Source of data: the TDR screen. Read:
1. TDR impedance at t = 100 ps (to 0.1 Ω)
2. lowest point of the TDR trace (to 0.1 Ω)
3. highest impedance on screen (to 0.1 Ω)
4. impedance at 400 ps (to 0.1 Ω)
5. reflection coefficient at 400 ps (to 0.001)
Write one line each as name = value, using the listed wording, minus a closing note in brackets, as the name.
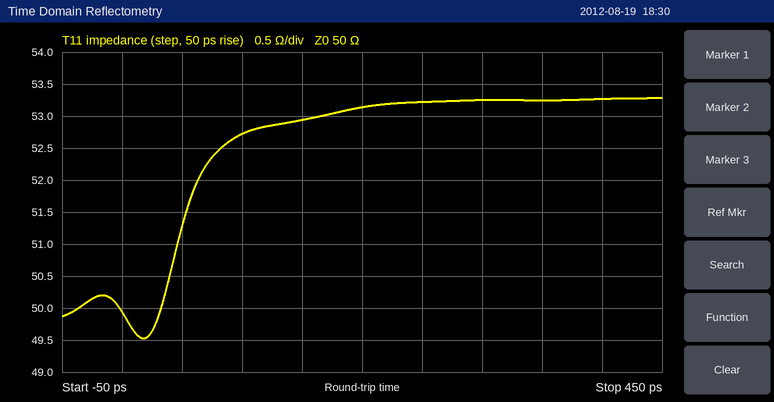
TDR impedance at t = 100 ps = 52.7 Ω
lowest point of the TDR trace = 49.5 Ω
highest impedance on screen = 53.3 Ω
impedance at 400 ps = 53.3 Ω
reflection coefficient at 400 ps = +0.032
